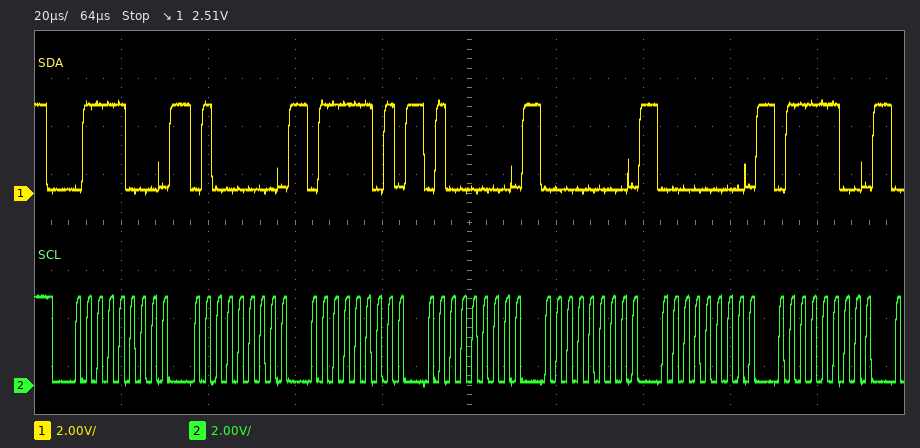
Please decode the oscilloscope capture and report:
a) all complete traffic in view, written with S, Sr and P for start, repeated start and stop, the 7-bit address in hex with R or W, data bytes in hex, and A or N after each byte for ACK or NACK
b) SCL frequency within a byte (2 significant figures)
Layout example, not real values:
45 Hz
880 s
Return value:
S 3CW A 40 A 7D A 40 A 00 A 00 A 7C A
400 kHz
